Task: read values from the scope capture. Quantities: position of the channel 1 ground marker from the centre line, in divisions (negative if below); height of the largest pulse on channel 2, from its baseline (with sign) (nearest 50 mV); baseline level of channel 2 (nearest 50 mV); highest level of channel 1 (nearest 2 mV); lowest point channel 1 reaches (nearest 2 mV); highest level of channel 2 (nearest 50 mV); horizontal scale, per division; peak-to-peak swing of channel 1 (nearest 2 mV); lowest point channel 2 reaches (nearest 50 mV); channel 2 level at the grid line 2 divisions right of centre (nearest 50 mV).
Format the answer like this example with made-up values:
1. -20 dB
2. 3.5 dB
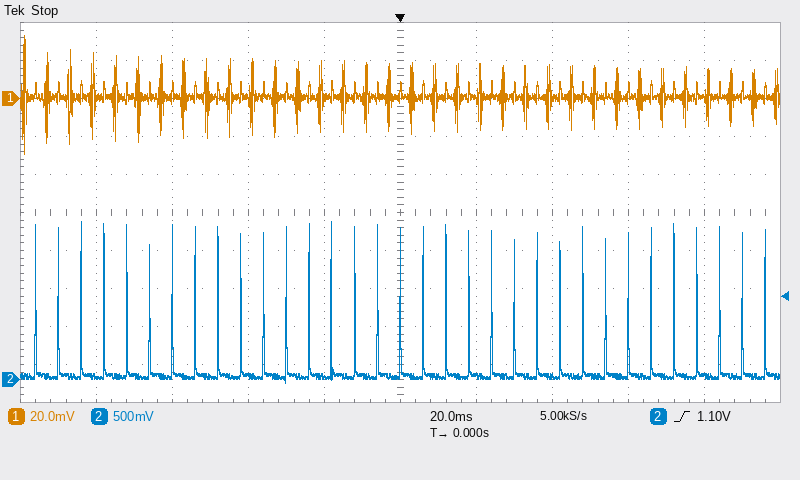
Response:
1. +3.0 div
2. +2.05 V
3. 50 mV
4. 34 mV
5. -28 mV
6. 2.10 V
7. 20 ms
8. 62 mV
9. -50 mV
10. 50 mV
